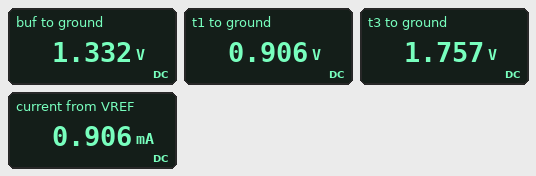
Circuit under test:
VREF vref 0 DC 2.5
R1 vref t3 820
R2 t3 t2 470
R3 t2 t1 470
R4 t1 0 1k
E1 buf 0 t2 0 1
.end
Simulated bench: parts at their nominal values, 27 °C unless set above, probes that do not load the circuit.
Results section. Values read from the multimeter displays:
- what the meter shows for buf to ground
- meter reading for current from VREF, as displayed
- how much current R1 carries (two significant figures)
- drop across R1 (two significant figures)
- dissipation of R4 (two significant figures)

1.332 V
0.906 mA
910 µA
740 mV
820 µW
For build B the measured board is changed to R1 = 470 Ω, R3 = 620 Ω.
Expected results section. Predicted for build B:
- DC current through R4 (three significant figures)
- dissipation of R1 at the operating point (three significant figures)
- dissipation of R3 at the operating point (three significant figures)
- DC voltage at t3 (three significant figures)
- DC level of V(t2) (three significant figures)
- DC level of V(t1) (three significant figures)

977 µA
448 µW
591 µW
2.04 V
1.58 V
977 mV
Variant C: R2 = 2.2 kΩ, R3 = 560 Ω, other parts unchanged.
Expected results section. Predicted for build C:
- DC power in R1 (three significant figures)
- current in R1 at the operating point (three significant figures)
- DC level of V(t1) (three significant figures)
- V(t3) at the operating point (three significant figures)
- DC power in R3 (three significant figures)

244 µW
546 µA
546 mV
2.05 V
167 µW
